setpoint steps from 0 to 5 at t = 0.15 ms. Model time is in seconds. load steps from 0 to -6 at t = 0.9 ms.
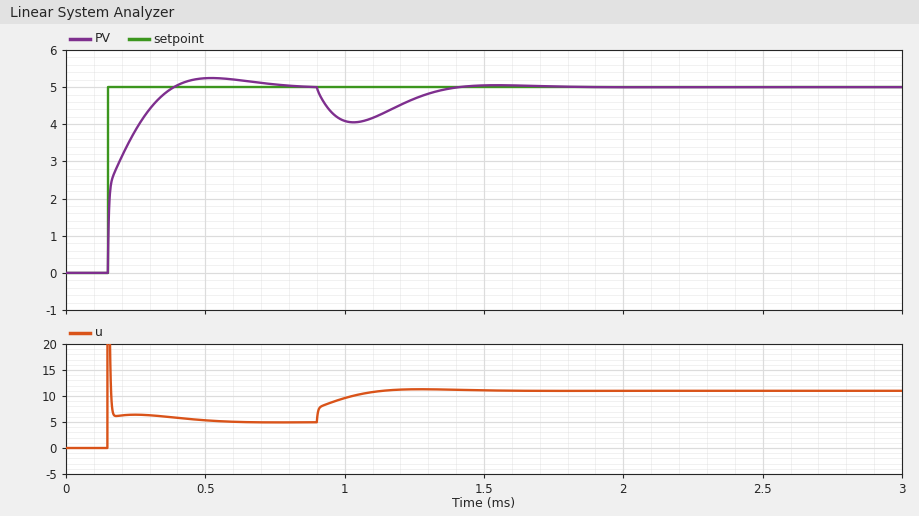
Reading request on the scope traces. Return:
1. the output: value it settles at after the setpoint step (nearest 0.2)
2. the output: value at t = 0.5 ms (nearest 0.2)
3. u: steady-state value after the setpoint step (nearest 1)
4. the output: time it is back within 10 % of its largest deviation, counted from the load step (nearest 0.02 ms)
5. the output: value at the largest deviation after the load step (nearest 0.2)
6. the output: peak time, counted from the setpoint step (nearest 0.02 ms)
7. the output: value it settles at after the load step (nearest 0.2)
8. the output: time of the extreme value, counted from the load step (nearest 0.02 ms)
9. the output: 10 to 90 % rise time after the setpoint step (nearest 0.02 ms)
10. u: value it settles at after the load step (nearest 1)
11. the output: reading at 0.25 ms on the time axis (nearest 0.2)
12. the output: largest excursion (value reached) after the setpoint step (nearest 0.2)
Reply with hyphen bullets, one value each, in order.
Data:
- 5.0
- 5.2
- 5
- 0.44 ms
- 4.0
- 0.38 ms
- 5.0
- 0.14 ms
- 0.16 ms
- 11
- 3.8
- 5.2
